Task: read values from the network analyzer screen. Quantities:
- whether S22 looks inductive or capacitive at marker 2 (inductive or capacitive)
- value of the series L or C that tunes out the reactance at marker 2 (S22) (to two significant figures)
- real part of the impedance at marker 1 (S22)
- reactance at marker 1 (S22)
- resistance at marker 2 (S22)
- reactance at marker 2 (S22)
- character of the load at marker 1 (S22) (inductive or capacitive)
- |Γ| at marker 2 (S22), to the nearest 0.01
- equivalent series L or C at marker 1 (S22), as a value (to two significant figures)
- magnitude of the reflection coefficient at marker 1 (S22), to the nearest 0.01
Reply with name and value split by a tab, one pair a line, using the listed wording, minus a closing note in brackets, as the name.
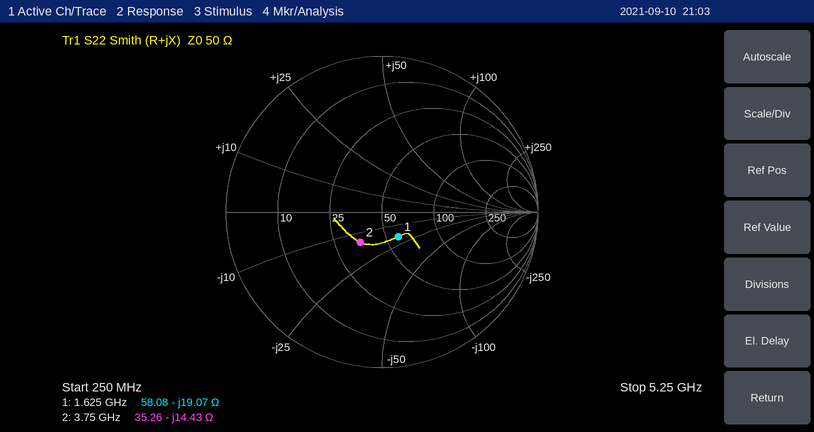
whether S22 looks inductive or capacitive at marker 2	capacitive
value of the series L or C that tunes out the reactance at marker 2 (S22)	610 pH
real part of the impedance at marker 1	58.08 Ω
reactance at marker 1	-19.07 Ω
resistance at marker 2	35.26 Ω
reactance at marker 2	-14.43 Ω
character of the load at marker 1 (S22)	capacitive
|Γ| at marker 2 (S22), to the nearest 0.01	0.24
equivalent series L or C at marker 1 (S22), as a value	5.1 pF
magnitude of the reflection coefficient at marker 1 (S22), to the nearest 0.01	0.19
